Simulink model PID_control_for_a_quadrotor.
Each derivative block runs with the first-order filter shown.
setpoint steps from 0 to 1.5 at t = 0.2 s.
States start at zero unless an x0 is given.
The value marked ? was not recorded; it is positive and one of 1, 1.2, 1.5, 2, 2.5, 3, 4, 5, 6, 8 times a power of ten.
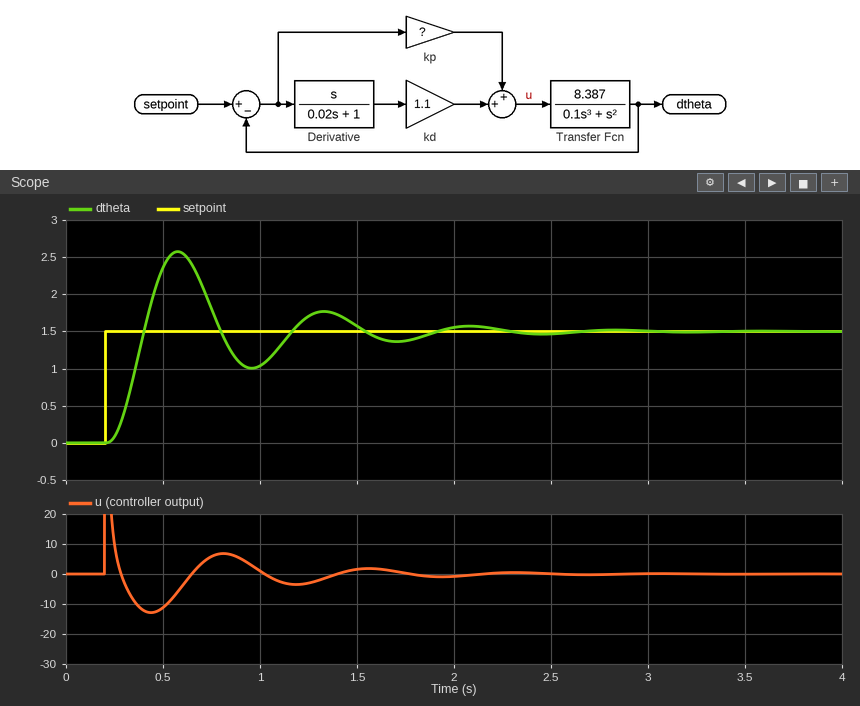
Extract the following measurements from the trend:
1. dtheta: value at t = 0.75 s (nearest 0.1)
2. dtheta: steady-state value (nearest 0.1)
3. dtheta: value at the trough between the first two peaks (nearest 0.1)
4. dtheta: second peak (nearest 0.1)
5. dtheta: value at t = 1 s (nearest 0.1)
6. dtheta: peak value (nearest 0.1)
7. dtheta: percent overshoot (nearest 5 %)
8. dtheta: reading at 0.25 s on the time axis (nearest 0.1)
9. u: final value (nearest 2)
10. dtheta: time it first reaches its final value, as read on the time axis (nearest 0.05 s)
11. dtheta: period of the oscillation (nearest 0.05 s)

1.8
1.5
1.0
1.8
1.0
2.6
70 %
0.1
0
0.40 s
0.75 s
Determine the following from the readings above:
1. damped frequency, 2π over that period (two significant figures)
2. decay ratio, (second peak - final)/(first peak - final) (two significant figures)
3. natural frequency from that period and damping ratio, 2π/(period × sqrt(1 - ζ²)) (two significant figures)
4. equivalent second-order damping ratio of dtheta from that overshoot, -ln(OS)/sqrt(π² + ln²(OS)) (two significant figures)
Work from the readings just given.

8.4 rad/s
0.27
8.4 rad/s
0.11
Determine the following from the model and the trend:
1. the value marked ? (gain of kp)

4
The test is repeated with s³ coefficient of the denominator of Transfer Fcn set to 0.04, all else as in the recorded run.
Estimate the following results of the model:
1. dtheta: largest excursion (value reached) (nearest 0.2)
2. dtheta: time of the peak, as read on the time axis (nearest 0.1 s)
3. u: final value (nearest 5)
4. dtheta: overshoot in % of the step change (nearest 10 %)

2.2
0.5 s
0
40 %
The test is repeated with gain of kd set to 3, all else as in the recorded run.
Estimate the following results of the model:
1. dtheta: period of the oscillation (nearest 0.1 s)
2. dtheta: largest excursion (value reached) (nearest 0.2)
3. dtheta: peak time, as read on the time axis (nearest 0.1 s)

0.4 s
2.6
0.4 s
